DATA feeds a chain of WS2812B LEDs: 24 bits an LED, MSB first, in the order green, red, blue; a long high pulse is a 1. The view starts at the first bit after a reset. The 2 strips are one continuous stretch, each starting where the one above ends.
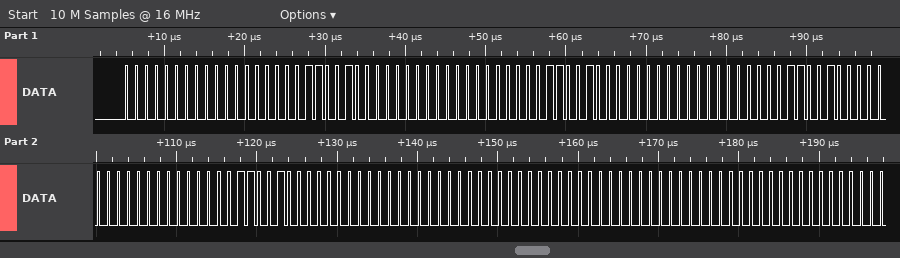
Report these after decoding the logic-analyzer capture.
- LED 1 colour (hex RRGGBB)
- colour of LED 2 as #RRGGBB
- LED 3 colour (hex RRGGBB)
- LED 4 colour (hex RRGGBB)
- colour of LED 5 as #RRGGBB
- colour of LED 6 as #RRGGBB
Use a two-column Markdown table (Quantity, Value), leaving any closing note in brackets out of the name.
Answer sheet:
| Quantity | Value |
|---|---|
| LED 1 colour | #000032 |
| colour of LED 2 as #RRGGBB | #000032 |
| LED 3 colour | #000032 |
| LED 4 colour | #000032 |
| colour of LED 5 as #RRGGBB | #000000 |
| colour of LED 6 as #RRGGBB | #000000 |
